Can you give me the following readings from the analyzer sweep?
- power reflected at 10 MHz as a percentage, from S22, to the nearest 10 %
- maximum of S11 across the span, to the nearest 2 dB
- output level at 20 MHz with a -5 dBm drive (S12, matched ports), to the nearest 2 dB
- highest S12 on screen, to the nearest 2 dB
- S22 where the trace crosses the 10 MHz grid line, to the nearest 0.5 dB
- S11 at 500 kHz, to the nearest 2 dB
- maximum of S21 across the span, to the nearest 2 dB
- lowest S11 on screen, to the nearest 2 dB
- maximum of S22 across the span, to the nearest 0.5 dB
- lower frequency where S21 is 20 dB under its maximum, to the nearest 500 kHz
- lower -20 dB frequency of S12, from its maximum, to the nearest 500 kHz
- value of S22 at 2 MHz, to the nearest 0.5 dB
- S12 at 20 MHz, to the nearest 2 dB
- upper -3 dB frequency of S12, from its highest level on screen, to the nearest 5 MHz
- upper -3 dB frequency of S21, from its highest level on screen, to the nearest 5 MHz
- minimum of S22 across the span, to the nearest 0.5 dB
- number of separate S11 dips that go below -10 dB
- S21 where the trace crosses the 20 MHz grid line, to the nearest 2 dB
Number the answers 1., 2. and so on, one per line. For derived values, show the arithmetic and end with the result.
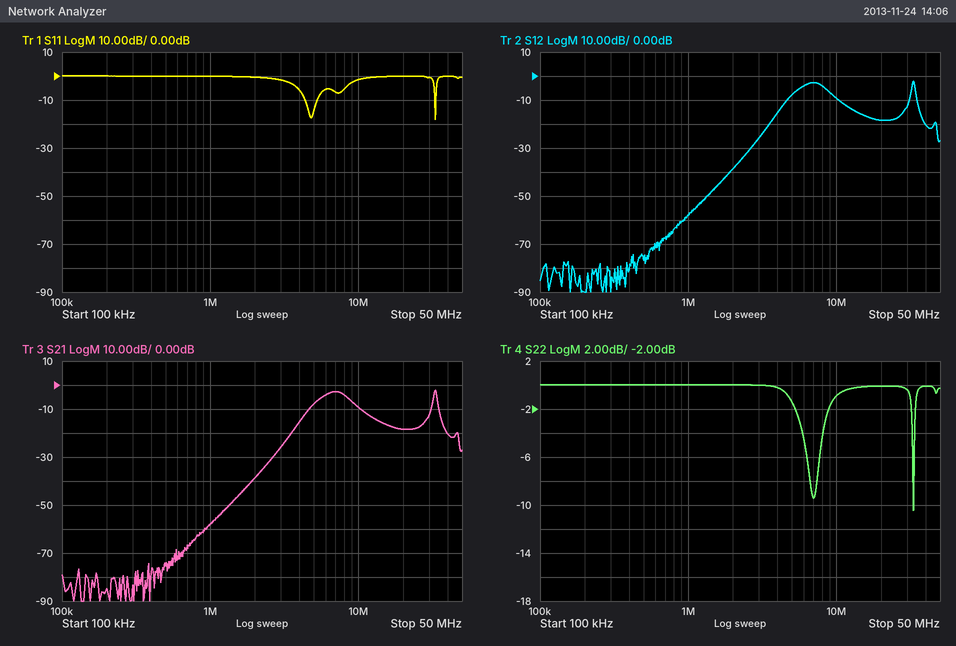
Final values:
1. 10^(-1/10) ≈ 79.4 %, so 80 % to the nearest 10 %
2. 0 dB
3. -5 dBm + (-18 dB) = -24 dBm
4. -2 dB
5. -1.0 dB
6. 0 dB
7. -2 dB
8. -18 dB
9. 0.0 dB
10. 3.5 MHz
11. 3.5 MHz
12. 0.0 dB
13. -18 dB
14. 35 MHz
15. 35 MHz
16. -10.5 dB
17. 2
18. -18 dB
